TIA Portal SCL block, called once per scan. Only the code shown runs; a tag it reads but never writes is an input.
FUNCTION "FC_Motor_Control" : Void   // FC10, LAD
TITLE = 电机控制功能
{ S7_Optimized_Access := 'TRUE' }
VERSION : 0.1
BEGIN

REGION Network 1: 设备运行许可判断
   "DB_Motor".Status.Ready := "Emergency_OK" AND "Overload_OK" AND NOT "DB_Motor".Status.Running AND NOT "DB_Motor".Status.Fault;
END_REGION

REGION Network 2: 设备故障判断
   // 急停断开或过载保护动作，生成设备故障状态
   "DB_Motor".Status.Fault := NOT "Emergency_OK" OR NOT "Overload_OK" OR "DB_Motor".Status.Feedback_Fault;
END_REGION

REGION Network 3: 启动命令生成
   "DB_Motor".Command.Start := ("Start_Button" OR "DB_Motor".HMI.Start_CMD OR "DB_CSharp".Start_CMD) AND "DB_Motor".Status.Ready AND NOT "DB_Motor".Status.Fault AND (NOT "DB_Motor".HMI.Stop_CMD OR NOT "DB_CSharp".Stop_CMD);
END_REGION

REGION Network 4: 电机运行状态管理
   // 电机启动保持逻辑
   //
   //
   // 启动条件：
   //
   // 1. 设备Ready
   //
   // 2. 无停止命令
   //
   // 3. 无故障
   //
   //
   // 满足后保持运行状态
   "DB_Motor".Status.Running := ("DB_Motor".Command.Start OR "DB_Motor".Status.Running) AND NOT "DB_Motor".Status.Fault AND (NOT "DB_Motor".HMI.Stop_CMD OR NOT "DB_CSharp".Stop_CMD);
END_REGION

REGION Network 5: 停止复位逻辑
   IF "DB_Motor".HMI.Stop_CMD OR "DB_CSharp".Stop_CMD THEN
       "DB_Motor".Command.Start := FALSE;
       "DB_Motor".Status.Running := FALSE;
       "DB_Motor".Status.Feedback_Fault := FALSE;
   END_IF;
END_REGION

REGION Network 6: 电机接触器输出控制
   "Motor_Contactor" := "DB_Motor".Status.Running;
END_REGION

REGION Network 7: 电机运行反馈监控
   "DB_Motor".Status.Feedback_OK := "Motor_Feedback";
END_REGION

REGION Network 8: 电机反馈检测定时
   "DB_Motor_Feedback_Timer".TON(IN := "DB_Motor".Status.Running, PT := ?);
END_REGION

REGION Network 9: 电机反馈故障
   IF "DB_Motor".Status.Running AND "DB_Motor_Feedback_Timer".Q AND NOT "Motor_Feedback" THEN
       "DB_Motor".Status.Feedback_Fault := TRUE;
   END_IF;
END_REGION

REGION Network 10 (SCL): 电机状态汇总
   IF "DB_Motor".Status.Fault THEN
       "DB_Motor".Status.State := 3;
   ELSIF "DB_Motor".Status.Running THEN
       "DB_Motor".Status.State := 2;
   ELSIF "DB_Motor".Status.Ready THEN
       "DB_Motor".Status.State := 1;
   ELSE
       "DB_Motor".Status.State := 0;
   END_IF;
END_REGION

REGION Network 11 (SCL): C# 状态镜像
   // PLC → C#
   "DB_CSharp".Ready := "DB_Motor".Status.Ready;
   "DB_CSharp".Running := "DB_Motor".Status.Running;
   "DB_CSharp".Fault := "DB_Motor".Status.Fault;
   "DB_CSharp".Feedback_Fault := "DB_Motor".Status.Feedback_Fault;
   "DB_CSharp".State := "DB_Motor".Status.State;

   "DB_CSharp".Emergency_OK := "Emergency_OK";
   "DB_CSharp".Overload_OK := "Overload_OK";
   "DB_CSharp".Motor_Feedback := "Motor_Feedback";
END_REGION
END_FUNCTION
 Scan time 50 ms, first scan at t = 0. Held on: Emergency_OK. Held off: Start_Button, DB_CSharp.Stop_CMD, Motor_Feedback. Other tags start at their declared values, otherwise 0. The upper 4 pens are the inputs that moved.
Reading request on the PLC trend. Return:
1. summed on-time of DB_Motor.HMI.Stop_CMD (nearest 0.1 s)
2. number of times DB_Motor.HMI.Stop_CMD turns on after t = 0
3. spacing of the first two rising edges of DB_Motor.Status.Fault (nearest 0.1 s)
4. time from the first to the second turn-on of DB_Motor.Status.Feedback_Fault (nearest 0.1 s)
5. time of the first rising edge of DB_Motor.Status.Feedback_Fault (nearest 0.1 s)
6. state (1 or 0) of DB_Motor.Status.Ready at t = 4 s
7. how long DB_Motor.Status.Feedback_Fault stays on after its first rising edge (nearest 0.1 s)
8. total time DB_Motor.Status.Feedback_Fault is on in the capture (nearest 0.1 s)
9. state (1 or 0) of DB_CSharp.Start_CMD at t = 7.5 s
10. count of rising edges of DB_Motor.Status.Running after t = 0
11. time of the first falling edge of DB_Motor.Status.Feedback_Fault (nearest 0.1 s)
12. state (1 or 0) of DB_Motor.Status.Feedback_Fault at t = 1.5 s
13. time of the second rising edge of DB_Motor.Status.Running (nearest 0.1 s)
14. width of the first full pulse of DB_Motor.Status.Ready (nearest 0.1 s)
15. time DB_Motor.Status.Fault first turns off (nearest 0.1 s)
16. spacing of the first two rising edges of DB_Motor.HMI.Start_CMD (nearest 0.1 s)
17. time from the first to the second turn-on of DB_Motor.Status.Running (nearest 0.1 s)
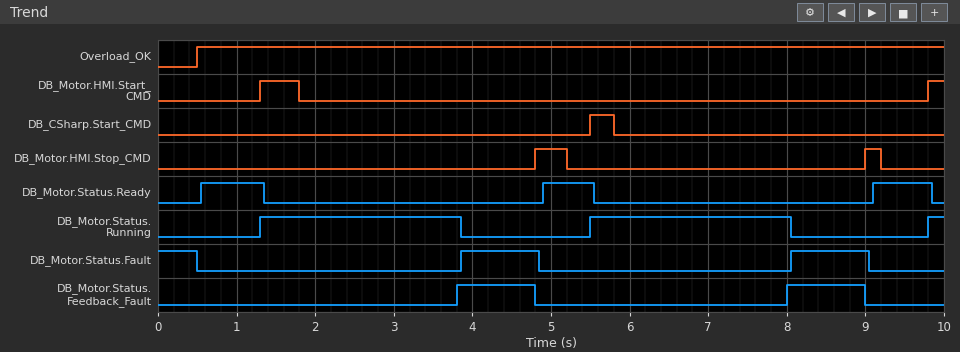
0.6 s
2
4.2 s
4.2 s
3.8 s
0
1.0 s
2.0 s
0
3
4.8 s
0
5.5 s
0.8 s
0.5 s
8.5 s
4.2 s
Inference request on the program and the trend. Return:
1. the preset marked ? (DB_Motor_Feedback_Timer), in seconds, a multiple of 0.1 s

2.5 s
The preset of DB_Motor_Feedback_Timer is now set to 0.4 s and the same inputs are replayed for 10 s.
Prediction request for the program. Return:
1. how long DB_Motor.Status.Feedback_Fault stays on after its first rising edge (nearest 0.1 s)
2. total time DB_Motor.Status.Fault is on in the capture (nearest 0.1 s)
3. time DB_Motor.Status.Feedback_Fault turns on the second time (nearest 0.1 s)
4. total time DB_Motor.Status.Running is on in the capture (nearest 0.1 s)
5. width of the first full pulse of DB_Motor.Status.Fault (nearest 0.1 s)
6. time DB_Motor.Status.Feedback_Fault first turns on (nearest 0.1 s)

3.1 s
6.7 s
5.9 s
1.1 s
3.1 s
1.7 s
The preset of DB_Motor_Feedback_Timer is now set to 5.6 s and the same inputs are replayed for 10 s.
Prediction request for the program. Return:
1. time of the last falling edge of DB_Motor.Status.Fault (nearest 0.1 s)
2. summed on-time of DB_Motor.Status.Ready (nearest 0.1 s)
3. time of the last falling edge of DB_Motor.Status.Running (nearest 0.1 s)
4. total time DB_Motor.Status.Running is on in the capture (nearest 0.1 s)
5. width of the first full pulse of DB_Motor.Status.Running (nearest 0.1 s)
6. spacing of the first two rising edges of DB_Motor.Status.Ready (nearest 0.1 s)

0.5 s
2.3 s
9.0 s
7.2 s
3.5 s
4.3 s
